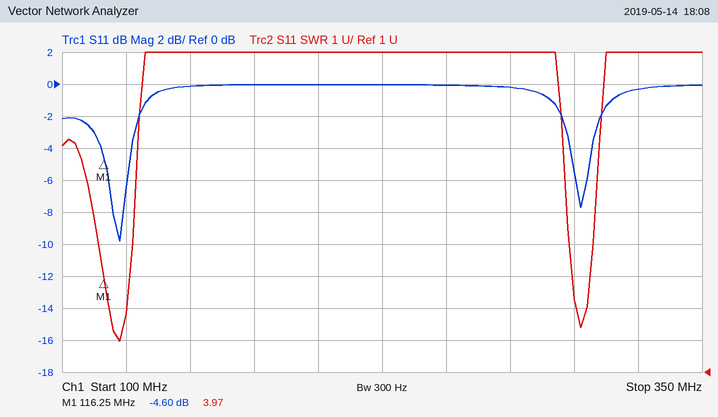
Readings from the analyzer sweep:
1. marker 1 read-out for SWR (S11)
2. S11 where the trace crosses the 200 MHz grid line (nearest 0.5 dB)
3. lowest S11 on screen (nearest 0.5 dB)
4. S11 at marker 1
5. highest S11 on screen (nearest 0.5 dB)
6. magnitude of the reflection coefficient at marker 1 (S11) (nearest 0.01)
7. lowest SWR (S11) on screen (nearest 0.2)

3.97
0.0 dB
-10.0 dB
-4.60 dB
0.0 dB
0.59
2.0
